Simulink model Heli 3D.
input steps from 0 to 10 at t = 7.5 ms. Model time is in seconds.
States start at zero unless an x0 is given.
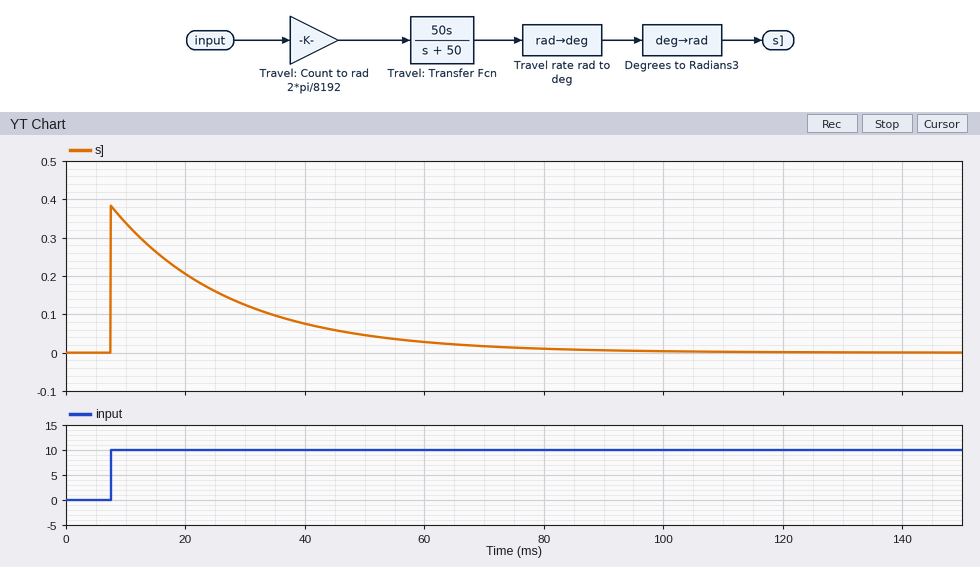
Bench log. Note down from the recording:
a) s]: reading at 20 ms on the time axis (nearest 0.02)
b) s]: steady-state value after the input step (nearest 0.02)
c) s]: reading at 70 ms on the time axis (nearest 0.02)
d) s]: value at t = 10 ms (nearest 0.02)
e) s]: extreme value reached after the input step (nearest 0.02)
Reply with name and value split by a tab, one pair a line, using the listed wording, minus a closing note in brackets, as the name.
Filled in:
s]: reading at 20 ms on the time axis	0.20
s]: steady-state value after the input step	0.00
s]: reading at 70 ms on the time axis	0.02
s]: value at t = 10 ms	0.34
s]: extreme value reached after the input step	0.38
